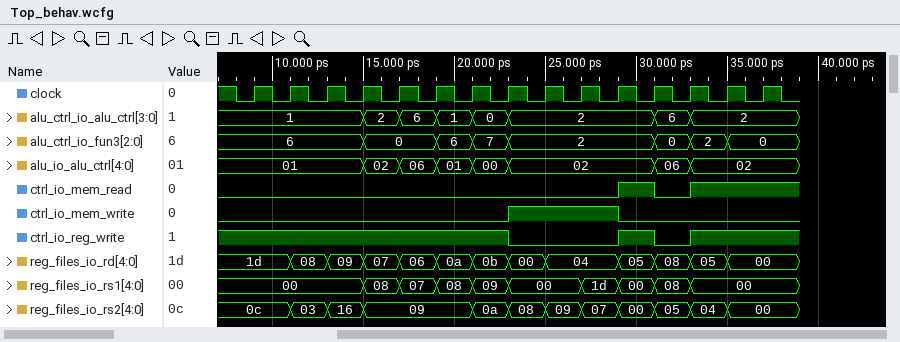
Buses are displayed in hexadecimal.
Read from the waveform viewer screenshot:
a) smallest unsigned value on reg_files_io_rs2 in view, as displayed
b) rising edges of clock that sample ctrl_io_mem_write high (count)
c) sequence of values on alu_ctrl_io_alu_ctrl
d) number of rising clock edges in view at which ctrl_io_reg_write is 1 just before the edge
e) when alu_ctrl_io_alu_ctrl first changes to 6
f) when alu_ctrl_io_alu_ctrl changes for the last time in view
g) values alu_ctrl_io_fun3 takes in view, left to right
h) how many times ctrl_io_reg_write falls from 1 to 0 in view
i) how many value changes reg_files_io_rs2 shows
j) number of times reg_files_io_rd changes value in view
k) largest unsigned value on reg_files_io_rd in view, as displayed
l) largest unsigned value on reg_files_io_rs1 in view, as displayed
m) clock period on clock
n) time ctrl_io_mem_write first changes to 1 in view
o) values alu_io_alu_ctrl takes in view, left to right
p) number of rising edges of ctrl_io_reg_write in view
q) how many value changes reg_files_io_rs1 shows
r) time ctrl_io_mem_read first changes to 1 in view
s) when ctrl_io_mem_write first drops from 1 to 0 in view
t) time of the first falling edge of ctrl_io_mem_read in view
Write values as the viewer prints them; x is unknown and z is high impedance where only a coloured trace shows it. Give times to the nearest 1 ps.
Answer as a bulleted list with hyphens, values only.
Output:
- 00
- 3
- 1, 2, 6, 1, 0, 2, 6, 2
- 11
- 17 ps
- 33 ps
- 6, 0, 6, 7, 2, 0, 2, 0
- 2
- 11
- 12
- 1d
- 1d
- 2 ps
- 23 ps
- 01, 02, 06, 01, 00, 02, 06, 02
- 2
- 9
- 29 ps
- 29 ps
- 31 ps
